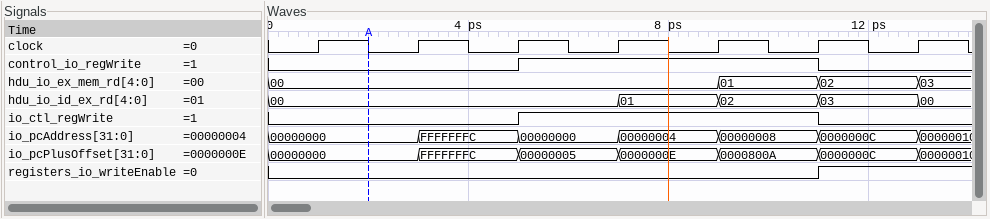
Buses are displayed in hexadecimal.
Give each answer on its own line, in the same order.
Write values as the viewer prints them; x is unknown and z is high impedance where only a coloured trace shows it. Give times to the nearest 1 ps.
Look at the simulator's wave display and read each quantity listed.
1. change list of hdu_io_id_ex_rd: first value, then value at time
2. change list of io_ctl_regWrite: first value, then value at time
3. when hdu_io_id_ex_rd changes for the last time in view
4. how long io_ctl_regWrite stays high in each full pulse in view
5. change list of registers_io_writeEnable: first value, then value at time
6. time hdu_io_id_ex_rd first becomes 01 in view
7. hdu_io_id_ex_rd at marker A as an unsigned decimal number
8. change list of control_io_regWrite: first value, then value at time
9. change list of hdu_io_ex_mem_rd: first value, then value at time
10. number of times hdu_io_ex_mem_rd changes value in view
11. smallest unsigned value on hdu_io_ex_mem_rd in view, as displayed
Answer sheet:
00, 01 at 7 ps, 02 at 9 ps, 03 at 11 ps, 00 at 13 ps
0, 1 at 5 ps, 0 at 11 ps
13 ps
6 ps
0, 1 at 11 ps
7 ps
0
0, 1 at 5 ps, 0 at 11 ps
00, 01 at 9 ps, 02 at 11 ps, 03 at 13 ps
3
00
